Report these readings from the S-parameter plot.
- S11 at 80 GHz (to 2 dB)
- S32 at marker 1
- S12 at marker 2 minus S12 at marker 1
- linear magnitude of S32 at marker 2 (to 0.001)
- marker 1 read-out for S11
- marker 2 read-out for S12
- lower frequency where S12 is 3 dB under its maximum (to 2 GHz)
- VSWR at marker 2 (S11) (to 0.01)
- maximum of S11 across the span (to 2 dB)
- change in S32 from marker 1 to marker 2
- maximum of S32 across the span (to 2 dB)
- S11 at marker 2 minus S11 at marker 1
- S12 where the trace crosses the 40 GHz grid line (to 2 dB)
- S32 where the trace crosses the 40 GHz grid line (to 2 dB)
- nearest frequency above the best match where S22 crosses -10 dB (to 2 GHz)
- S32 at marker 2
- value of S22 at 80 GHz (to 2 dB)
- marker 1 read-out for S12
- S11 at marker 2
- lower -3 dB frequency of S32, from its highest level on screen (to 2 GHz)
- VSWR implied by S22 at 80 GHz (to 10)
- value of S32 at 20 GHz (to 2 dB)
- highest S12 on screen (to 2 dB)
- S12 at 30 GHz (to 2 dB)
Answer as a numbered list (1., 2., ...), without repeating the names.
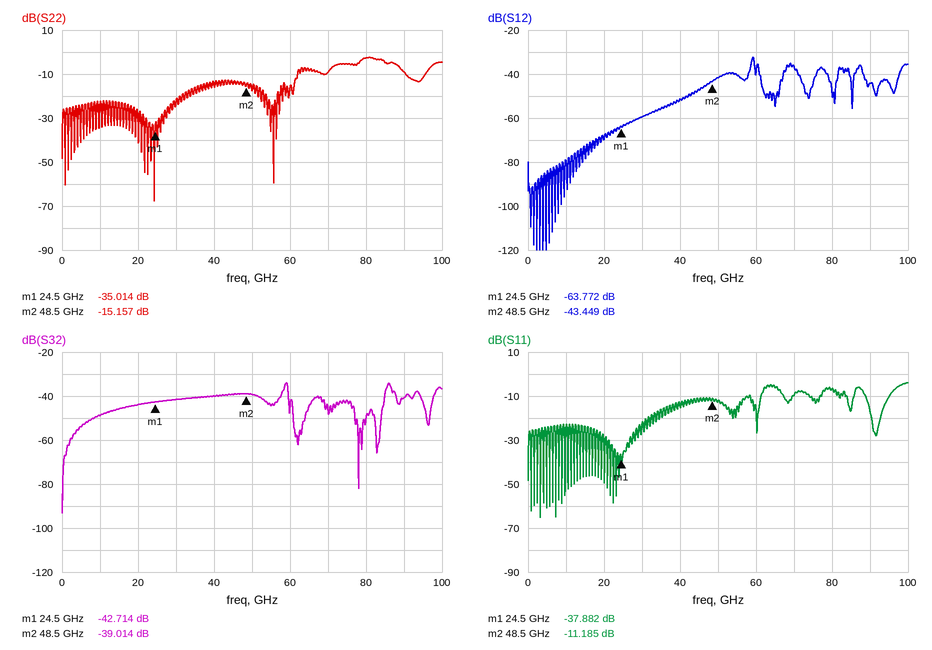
1. -6 dB
2. -42.714 dB
3. 20.323 dB
4. 0.011
5. -37.882 dB
6. -43.449 dB
7. 58 GHz
8. 1.76
9. -4 dB
10. 3.700 dB
11. -34 dB
12. 26.697 dB
13. -52 dB
14. -40 dB
15. 62 GHz
16. -39.014 dB
17. -2 dB
18. -63.772 dB
19. -11.185 dB
20. 58 GHz
21. 10
22. -44 dB
23. -32 dB
24. -60 dB
